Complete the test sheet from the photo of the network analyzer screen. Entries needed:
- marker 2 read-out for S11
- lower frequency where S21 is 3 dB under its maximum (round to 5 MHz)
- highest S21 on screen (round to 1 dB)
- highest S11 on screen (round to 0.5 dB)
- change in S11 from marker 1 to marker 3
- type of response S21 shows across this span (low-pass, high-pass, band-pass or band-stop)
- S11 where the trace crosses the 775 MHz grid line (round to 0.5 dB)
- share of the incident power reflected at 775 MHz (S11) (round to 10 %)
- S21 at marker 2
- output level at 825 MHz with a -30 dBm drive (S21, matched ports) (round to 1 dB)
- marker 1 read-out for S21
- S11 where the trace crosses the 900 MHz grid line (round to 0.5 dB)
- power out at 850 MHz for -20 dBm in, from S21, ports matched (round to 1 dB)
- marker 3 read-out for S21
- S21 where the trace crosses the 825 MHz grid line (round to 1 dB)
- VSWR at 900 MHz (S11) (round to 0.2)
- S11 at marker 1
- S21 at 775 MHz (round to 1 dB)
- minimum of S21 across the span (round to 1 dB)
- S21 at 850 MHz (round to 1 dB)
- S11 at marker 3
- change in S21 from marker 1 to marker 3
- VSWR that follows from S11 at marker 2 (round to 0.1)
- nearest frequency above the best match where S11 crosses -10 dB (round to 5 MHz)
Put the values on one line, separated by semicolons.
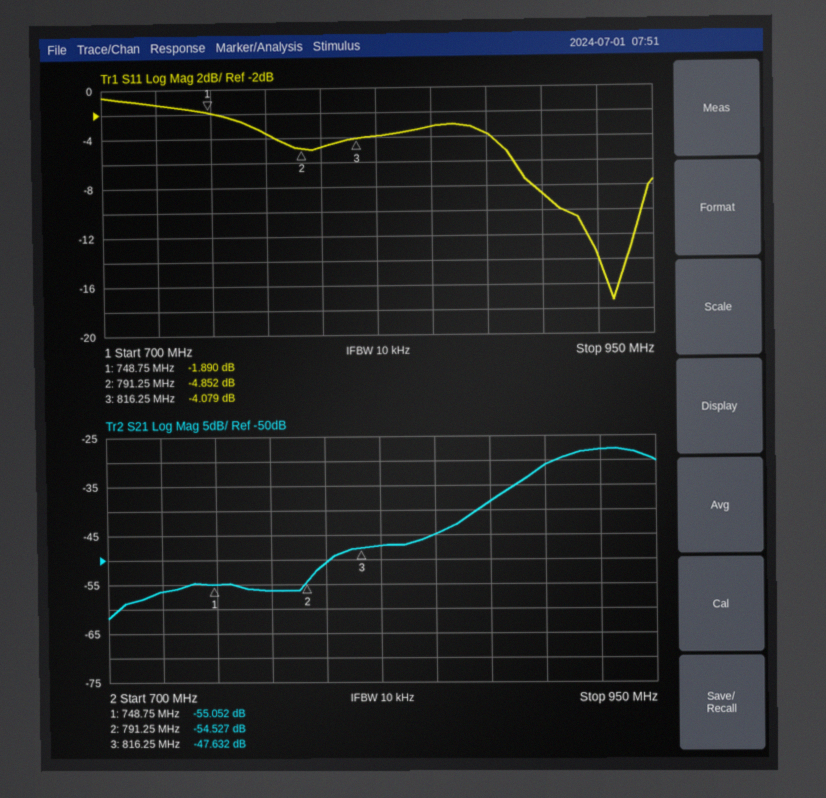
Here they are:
-4.852 dB; 900 MHz; -28 dB; -0.5 dB; -2.189 dB; high-pass; -3.5 dB; 40 %; -54.527 dB; -77 dBm; -55.052 dB; -8.5 dB; -65 dBm; -47.632 dB; -47 dB; 2.2; -1.890 dB; -56 dB; -62 dB; -45 dB; -4.079 dB; 7.420 dB; 3.7; 945 MHz
